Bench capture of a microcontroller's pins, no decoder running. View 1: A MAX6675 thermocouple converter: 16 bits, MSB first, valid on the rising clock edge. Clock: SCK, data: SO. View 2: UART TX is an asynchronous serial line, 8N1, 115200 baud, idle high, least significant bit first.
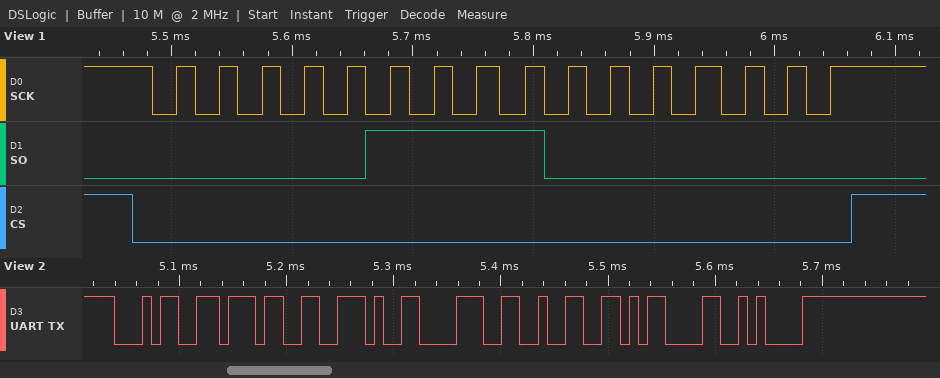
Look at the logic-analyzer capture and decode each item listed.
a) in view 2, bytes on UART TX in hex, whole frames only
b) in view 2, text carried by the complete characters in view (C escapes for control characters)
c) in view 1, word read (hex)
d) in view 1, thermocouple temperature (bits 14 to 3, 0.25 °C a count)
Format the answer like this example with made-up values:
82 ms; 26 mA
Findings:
34 37 2E 38 32 0D 0A; "47.82\r\n"; 0x0780; 60.00 °C
